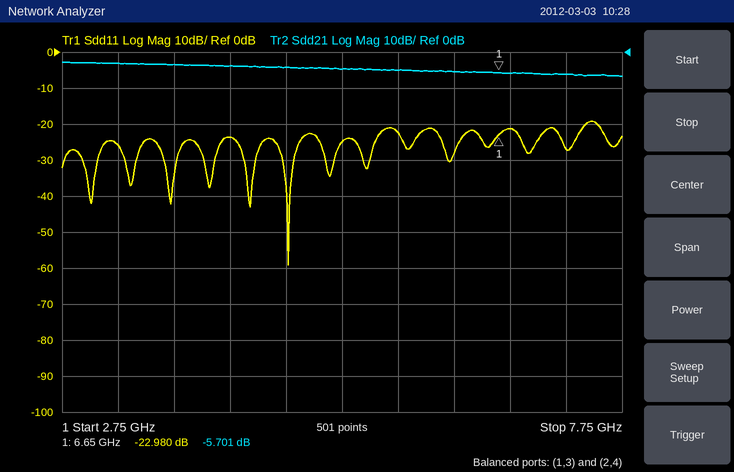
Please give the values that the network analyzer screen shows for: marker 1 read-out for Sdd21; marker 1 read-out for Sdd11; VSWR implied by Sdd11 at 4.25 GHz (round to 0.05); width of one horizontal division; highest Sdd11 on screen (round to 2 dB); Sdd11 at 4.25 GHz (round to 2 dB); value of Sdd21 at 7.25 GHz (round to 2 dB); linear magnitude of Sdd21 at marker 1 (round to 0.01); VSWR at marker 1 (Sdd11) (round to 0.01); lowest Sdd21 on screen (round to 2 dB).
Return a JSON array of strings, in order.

["-5.701 dB", "-22.980 dB", "1.15", "500 MHz", "-20 dB", "-24 dB", "-6 dB", "0.52", "1.15", "-6 dB"]
